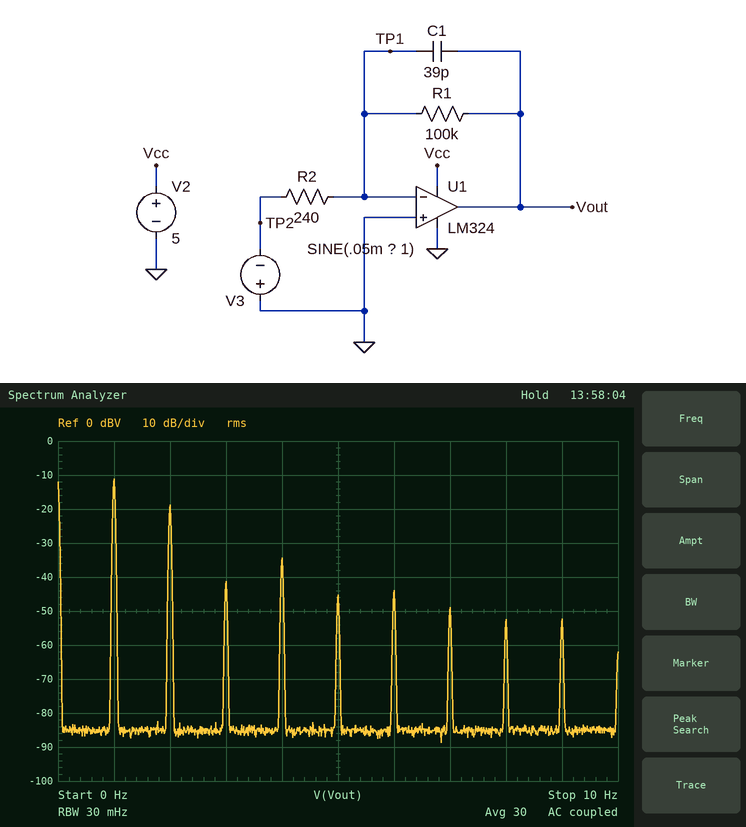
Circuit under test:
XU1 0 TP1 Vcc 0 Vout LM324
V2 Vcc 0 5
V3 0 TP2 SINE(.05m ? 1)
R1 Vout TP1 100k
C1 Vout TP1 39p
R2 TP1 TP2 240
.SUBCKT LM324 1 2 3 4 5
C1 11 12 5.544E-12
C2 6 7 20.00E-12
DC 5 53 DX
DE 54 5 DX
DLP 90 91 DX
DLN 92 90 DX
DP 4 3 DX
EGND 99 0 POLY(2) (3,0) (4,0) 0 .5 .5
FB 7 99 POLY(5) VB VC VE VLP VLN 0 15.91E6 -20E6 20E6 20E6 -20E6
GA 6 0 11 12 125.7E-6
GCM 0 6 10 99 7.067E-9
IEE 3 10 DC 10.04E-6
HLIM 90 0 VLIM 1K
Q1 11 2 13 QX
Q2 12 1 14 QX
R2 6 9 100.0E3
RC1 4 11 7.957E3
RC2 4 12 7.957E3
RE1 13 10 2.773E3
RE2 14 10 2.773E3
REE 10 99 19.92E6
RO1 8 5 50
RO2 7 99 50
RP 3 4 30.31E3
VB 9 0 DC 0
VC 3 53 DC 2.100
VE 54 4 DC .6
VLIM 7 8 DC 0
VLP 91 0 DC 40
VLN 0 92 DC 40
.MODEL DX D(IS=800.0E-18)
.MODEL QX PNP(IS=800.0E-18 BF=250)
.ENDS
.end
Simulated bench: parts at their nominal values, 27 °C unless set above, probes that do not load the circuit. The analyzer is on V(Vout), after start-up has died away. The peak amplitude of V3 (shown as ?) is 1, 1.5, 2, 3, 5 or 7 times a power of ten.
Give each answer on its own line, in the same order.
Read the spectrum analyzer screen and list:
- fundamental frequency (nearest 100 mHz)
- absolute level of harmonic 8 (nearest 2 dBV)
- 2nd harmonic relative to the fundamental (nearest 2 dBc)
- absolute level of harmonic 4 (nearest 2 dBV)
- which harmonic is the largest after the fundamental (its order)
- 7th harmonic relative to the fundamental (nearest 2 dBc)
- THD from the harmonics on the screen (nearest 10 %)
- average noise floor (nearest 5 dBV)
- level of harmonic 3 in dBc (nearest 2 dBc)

1.0 Hz
-52 dBV
-8 dBc
-34 dBV
2
-38 dBc
40 %
-85 dBV
-30 dBc
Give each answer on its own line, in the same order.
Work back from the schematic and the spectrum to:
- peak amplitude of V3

2 mV
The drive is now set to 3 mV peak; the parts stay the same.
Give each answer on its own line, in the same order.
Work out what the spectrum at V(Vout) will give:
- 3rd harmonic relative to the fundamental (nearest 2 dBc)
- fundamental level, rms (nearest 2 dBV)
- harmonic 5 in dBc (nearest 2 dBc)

-34 dBc
-8 dBV
-38 dBc
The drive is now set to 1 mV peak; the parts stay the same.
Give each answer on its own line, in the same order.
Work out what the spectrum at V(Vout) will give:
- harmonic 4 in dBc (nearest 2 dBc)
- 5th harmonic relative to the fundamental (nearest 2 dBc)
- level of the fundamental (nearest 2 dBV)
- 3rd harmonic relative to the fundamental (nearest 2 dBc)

-28 dBc
-30 dBc
-18 dBV
-24 dBc
